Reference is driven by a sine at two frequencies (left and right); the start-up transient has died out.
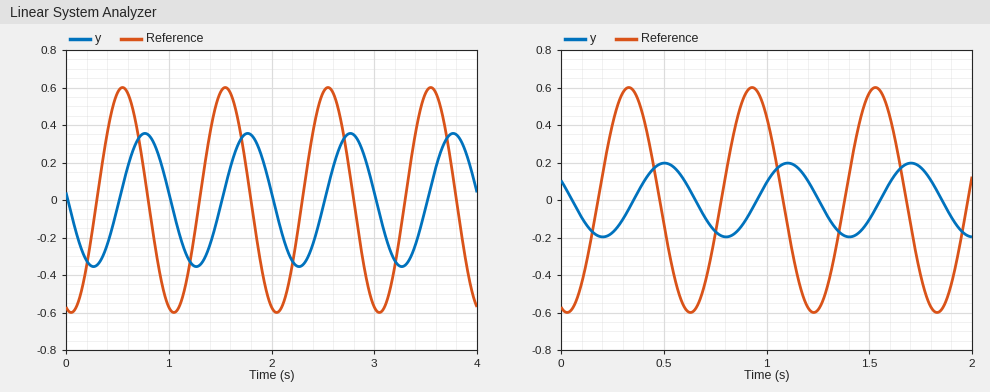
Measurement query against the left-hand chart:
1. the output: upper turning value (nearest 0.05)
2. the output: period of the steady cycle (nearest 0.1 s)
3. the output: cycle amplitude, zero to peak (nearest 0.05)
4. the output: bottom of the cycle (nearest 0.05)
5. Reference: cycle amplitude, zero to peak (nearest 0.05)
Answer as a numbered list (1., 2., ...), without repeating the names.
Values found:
1. 0.35
2. 1.0 s
3. 0.35
4. -0.35
5. 0.60
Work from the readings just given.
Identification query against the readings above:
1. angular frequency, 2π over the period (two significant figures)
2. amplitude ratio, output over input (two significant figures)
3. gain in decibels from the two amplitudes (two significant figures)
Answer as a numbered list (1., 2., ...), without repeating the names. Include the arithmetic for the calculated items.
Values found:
1. 2π / 1 = 6.3 rad/s
2. 0.35 / 0.6 = 0.58
3. 20 log10(0.35 / 0.6) = -4.7 dB
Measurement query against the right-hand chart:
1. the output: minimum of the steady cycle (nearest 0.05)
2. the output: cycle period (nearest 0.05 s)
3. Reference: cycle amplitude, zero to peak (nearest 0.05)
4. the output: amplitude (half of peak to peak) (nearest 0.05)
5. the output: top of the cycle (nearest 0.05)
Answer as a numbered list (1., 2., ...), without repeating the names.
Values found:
1. -0.20
2. 0.60 s
3. 0.60
4. 0.20
5. 0.20
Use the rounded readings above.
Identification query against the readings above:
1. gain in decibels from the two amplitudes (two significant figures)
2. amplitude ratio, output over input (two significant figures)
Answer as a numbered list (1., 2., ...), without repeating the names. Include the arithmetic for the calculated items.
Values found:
1. 20 log10(0.2 / 0.6) = -9.5 dB
2. 0.2 / 0.6 = 0.33
